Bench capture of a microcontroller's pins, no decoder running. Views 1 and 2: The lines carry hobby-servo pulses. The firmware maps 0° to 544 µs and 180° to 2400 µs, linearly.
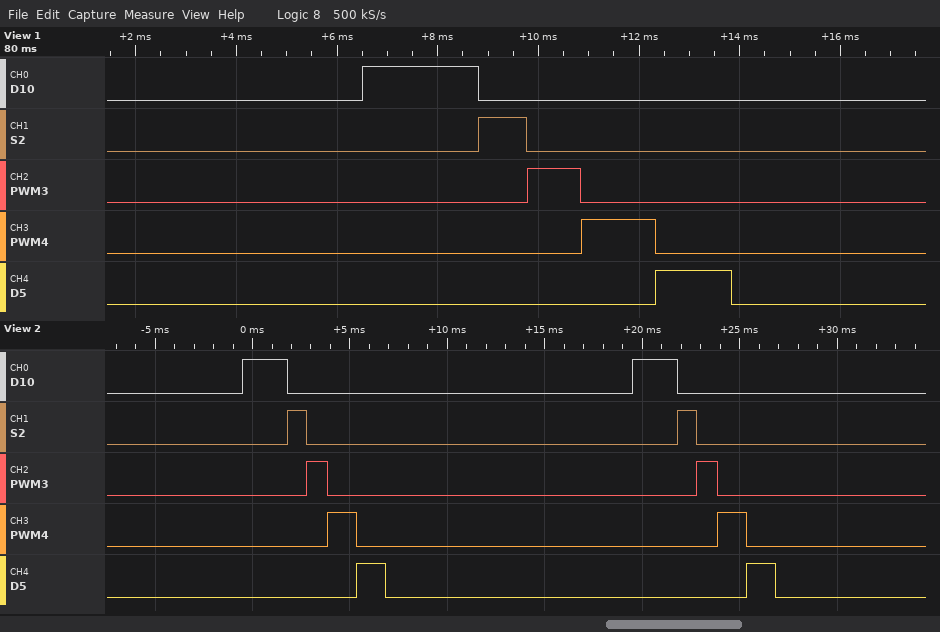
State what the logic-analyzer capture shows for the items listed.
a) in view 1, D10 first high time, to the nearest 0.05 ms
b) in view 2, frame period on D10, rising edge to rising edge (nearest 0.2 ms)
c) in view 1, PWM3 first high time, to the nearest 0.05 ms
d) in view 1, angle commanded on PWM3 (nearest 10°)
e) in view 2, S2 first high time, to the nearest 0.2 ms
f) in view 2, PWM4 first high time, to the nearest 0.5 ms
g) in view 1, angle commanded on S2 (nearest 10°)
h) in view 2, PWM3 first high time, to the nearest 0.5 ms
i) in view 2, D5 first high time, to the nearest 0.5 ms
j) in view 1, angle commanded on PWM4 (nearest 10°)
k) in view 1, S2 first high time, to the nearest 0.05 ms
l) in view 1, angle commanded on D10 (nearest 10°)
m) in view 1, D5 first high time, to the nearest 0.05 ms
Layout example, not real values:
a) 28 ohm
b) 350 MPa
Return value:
a) 2.30 ms
b) 20.0 ms
c) 1.05 ms
d) 50°
e) 1.0 ms
f) 1.5 ms
g) 40°
h) 1.0 ms
i) 1.5 ms
j) 90°
k) 0.95 ms
l) 170°
m) 1.50 ms
